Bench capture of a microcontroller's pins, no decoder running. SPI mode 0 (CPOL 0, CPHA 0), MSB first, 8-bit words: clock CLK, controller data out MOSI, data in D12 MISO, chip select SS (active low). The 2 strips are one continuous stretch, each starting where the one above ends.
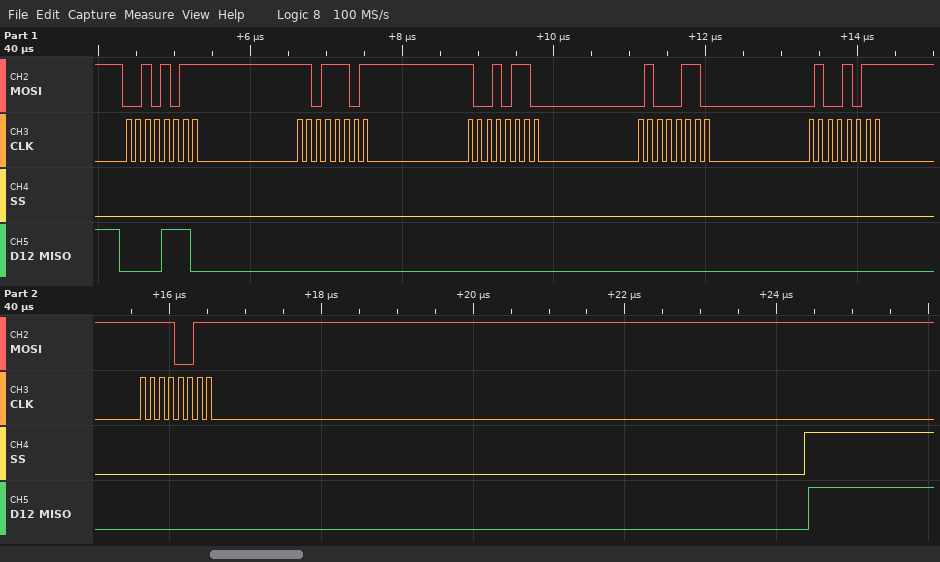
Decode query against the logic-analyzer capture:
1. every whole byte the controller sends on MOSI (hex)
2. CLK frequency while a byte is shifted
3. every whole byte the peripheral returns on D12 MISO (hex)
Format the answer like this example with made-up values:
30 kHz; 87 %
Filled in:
2B DD 96 46 4B F3; 8 MHz; 0E 00 00 00 00 00
